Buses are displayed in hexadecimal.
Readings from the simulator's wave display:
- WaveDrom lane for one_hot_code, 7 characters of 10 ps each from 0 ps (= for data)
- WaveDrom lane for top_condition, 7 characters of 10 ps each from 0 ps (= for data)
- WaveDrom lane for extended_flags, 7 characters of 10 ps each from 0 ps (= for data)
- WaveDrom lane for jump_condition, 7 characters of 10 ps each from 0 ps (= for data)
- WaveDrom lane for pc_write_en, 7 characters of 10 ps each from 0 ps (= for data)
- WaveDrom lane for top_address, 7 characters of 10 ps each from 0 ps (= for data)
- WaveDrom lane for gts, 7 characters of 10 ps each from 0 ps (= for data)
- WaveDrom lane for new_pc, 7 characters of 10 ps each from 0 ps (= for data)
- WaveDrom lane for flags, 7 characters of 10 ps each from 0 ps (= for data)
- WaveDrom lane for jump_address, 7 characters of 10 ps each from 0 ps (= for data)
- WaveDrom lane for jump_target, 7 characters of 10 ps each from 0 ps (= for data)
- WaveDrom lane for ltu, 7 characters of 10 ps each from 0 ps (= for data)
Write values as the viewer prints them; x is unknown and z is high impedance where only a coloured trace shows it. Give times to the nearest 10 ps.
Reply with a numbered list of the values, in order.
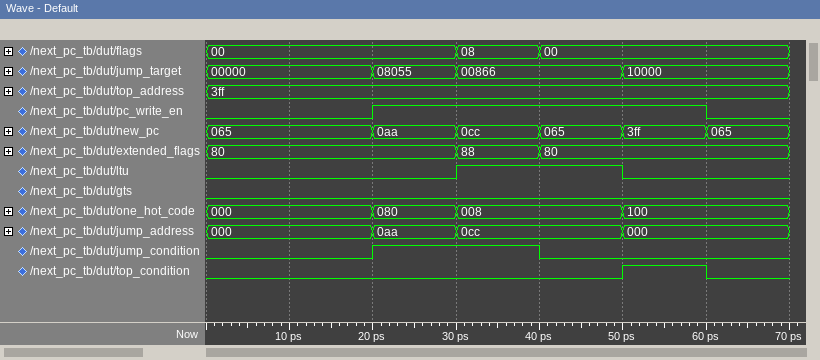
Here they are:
1. {name: 'one_hot_code', wave: '=.==.=.', data: '000 080 008 100'}
2. {name: 'top_condition', wave: '0....10'}
3. {name: 'extended_flags', wave: '=..==..', data: '80 88 80'}
4. {name: 'jump_condition', wave: '0.1.0..'}
5. {name: 'pc_write_en', wave: '0.1...0'}
6. {name: 'top_address', wave: '=......', data: '3ff'}
7. {name: 'gts', wave: '0......'}
8. {name: 'new_pc', wave: '=.=====', data: '065 0aa 0cc 065 3ff 065'}
9. {name: 'flags', wave: '=..==..', data: '00 08 00'}
10. {name: 'jump_address', wave: '=.==.=.', data: '000 0aa 0cc 000'}
11. {name: 'jump_target', wave: '=.==.=.', data: '00000 08055 00866 10000'}
12. {name: 'ltu', wave: '0..1.0.'}
